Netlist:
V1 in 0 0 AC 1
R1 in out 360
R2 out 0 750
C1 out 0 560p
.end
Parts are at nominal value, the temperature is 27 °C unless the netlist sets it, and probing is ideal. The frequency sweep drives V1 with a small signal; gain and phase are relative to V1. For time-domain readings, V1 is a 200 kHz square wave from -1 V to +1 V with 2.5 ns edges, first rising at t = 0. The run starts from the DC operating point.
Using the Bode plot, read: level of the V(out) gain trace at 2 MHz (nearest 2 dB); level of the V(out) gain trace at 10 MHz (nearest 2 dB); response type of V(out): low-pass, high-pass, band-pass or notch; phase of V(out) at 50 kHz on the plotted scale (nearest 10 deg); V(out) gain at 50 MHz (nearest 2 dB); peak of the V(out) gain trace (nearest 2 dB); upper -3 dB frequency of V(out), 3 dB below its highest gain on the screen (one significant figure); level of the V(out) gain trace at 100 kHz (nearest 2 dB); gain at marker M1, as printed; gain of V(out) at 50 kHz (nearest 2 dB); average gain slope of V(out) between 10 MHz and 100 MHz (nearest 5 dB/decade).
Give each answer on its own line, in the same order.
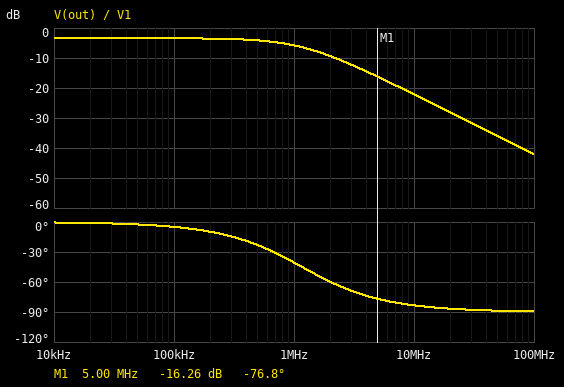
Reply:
-10 dB
-22 dB
low-pass
0 deg
-36 dB
-4 dB
1 MHz
-4 dB
-16.26 dB
-4 dB
-20 dB/decade
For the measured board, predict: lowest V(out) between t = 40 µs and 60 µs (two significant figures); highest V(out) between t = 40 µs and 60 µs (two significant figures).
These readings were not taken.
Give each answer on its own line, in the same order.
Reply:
-680 mV
680 mV
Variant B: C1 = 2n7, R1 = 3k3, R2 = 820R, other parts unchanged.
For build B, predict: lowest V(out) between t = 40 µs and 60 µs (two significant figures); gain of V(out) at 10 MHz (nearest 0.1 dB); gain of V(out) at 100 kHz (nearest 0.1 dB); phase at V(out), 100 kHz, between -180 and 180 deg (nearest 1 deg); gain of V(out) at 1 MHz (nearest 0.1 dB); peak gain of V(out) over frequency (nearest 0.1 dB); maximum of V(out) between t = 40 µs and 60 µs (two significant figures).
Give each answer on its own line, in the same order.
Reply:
-120 mV
-55.0 dB
-17.5 dB
-48 deg
-35.0 dB
-14.0 dB
120 mV
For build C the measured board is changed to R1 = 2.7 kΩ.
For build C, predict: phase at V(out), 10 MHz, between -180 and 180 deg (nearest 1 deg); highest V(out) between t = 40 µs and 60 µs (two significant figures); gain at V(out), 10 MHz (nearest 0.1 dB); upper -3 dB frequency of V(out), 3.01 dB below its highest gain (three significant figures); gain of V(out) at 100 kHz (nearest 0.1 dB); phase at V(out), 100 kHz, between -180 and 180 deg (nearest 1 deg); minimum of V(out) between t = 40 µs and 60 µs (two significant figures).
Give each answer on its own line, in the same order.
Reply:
-87 deg
220 mV
-39.6 dB
484 kHz
-13.4 dB
-12 deg
-220 mV
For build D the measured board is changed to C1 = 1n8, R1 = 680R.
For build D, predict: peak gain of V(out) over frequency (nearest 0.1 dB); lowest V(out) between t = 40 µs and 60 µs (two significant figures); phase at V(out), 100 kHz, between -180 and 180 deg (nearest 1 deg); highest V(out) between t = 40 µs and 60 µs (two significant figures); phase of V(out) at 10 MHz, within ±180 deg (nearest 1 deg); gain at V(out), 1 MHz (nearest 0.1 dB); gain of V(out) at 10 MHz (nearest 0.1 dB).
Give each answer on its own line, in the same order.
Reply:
-5.6 dB
-500 mV
-22 deg
500 mV
-89 deg
-18.0 dB
-37.7 dB
